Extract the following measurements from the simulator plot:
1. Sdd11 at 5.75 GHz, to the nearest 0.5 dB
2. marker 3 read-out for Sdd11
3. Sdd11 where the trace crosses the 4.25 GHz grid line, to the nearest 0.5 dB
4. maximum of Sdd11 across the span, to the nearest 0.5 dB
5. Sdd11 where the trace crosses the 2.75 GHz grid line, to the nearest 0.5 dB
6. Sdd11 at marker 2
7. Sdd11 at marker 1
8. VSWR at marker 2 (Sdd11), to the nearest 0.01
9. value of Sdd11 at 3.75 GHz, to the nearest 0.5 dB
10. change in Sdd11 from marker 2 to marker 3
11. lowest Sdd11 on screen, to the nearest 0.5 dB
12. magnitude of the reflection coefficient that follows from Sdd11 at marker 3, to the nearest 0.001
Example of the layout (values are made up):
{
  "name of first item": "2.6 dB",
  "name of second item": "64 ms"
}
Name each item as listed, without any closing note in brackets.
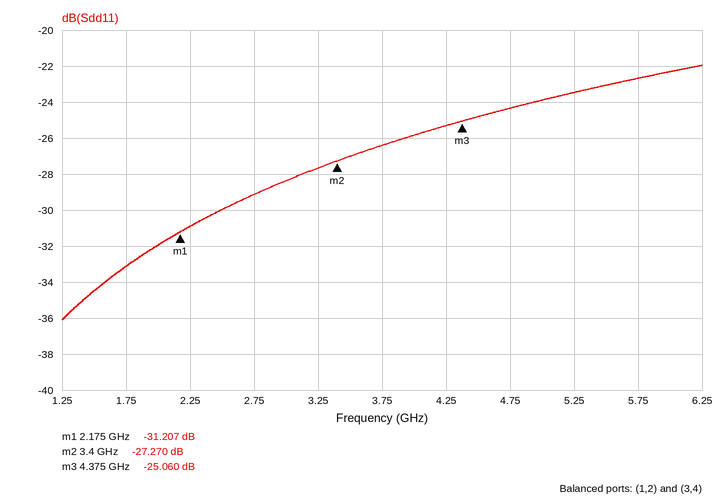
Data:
{
  "Sdd11 at 5.75 GHz, to the nearest 0.5 dB": "-22.5 dB",
  "marker 3 read-out for Sdd11": "-25.060 dB",
  "Sdd11 where the trace crosses the 4.25 GHz grid line, to the nearest 0.5 dB": "-25.5 dB",
  "maximum of Sdd11 across the span, to the nearest 0.5 dB": "-22.0 dB",
  "Sdd11 where the trace crosses the 2.75 GHz grid line, to the nearest 0.5 dB": "-29.0 dB",
  "Sdd11 at marker 2": "-27.270 dB",
  "Sdd11 at marker 1": "-31.207 dB",
  "VSWR at marker 2 (Sdd11), to the nearest 0.01": "1.09",
  "value of Sdd11 at 3.75 GHz, to the nearest 0.5 dB": "-26.5 dB",
  "change in Sdd11 from marker 2 to marker 3": "2.210 dB",
  "lowest Sdd11 on screen, to the nearest 0.5 dB": "-36.0 dB",
  "magnitude of the reflection coefficient that follows from Sdd11 at marker 3, to the nearest 0.001": "0.056"
}
